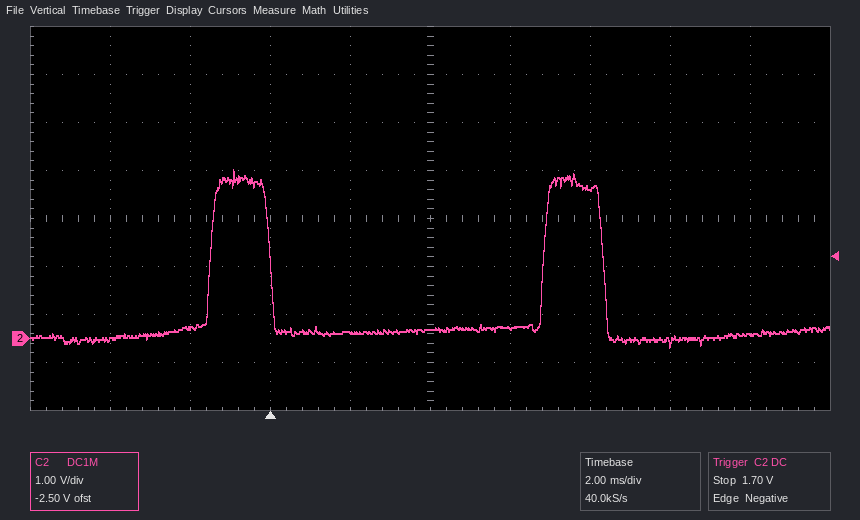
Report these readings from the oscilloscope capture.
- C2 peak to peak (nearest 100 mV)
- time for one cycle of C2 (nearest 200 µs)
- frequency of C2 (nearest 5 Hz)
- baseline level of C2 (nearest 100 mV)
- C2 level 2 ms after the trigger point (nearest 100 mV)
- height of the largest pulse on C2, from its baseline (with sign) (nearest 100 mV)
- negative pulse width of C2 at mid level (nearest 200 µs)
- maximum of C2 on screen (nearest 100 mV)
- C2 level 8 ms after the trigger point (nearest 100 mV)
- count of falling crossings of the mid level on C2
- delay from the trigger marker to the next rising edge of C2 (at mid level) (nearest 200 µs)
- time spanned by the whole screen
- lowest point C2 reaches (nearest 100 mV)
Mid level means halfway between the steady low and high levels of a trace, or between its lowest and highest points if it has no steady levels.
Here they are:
3.7 V
8.4 ms
120 Hz
100 mV
100 mV
+3.4 V
6.8 ms
3.5 V
3.1 V
2
6.8 ms
20 ms
-200 mV
